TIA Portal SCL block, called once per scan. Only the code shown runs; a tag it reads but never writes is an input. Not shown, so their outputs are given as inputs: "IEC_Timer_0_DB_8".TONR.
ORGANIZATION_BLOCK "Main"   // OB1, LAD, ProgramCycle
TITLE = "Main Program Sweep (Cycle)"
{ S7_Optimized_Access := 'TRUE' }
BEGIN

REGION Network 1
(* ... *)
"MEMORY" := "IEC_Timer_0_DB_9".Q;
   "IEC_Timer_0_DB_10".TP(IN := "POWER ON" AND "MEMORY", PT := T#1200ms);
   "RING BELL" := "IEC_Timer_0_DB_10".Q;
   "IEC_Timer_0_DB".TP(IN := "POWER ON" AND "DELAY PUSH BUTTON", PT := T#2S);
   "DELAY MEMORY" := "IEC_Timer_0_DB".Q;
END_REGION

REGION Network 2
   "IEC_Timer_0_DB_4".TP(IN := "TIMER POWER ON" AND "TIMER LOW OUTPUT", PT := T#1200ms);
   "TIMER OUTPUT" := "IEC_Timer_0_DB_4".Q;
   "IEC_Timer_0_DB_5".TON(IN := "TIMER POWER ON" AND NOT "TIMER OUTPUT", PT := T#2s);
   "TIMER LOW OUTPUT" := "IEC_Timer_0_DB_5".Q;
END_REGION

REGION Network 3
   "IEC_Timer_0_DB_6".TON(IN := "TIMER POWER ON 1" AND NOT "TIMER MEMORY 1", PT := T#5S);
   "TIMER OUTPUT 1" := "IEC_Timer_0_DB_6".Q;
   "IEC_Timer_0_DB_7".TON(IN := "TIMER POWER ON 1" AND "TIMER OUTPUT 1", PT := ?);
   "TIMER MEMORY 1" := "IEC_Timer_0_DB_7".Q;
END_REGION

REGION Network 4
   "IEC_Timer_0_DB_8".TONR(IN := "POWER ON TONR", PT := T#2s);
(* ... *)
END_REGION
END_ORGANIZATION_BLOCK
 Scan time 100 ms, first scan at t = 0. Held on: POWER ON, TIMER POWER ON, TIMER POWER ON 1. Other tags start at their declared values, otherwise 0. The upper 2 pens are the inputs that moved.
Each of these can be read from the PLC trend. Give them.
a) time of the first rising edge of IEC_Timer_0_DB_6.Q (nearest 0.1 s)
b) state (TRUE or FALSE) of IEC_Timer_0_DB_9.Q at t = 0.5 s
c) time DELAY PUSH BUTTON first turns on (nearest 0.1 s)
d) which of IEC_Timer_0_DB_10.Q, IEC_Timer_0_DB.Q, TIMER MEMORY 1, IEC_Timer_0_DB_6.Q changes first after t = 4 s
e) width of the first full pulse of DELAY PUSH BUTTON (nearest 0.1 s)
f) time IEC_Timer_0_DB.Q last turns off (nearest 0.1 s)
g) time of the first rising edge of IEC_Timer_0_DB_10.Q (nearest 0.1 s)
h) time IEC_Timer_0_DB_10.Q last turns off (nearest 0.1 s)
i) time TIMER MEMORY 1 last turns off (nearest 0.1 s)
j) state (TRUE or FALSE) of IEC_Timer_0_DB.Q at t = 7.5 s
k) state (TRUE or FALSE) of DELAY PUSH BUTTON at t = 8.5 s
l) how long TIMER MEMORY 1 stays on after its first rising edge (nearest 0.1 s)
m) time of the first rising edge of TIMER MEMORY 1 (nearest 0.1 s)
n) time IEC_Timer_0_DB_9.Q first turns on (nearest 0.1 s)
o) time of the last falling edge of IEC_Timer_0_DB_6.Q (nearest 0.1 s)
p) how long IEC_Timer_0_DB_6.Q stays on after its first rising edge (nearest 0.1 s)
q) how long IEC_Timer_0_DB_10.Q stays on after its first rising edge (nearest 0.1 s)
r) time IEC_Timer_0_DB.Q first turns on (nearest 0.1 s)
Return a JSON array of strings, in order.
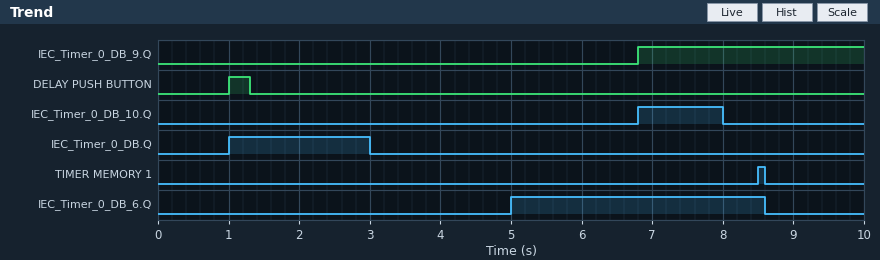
["5.0 s", "FALSE", "1.0 s", "IEC_Timer_0_DB_6.Q", "0.3 s", "3.0 s", "6.8 s", "8.0 s", "8.6 s", "FALSE", "FALSE", "0.1 s", "8.5 s", "6.8 s", "8.6 s", "3.6 s", "1.2 s", "1.0 s"]
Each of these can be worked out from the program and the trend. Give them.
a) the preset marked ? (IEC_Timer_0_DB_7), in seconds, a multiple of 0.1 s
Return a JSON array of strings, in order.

["3.5 s"]
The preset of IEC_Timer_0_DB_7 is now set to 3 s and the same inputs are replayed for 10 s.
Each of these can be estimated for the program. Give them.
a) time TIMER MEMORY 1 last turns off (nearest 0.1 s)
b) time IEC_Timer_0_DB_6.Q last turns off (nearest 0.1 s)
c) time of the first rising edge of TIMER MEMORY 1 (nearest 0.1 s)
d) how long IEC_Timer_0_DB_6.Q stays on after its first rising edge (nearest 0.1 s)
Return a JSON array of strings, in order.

["8.1 s", "8.1 s", "8.0 s", "3.1 s"]
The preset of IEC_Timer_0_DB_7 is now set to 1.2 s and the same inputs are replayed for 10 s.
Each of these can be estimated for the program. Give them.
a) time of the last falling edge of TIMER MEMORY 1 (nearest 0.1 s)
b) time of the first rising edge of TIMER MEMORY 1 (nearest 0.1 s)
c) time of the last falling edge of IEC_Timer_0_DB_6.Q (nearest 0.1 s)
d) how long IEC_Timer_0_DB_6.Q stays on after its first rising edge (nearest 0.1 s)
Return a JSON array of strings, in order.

["6.3 s", "6.2 s", "6.3 s", "1.3 s"]
